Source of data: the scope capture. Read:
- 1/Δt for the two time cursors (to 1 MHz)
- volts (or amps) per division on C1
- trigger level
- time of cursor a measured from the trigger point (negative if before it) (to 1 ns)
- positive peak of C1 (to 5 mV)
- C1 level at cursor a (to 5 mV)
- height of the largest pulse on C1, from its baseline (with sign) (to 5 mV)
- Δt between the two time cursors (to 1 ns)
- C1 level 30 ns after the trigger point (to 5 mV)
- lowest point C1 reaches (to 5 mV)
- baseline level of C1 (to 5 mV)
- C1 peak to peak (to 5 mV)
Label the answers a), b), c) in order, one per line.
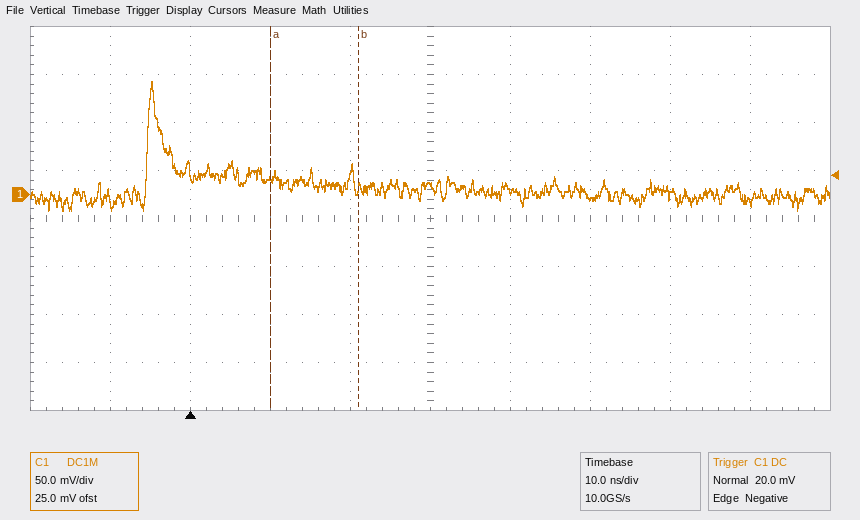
a) 91 MHz
b) 50 mV
c) 20.0 mV
d) +10 ns
e) 120 mV
f) 15 mV
g) +115 mV
h) 11 ns
i) 10 mV
j) -15 mV
k) 5 mV
l) 135 mV
